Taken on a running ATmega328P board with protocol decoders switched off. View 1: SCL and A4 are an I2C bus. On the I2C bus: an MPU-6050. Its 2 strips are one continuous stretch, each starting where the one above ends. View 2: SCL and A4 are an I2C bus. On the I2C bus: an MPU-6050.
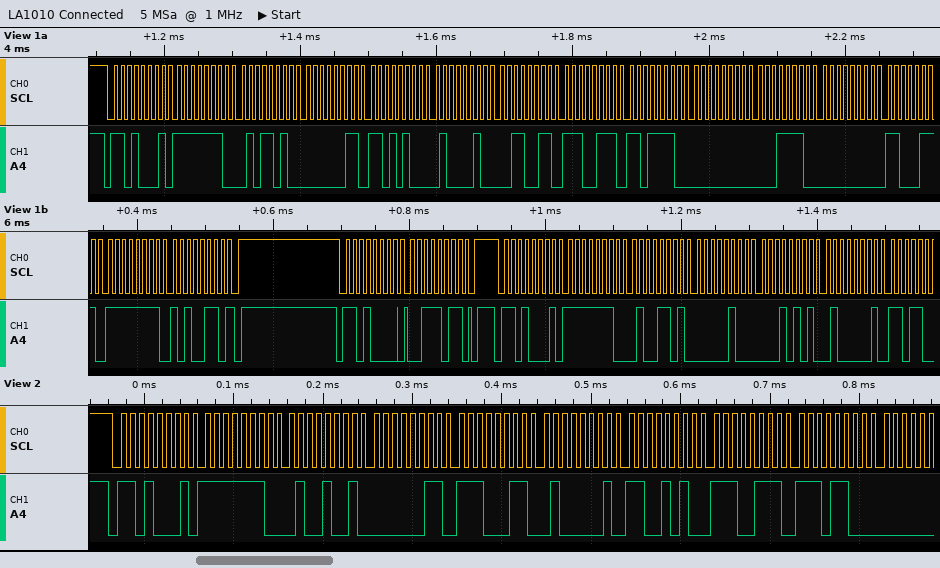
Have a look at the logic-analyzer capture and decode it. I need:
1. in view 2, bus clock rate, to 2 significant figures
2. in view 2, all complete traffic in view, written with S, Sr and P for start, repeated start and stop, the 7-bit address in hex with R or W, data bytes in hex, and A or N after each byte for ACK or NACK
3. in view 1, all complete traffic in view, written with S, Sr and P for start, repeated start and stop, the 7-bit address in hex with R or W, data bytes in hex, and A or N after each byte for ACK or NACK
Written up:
100 kHz
S 68R A FE A 49 A 03 A E3 A 41 A CA A E7 A EC A
S 68R A FE A 5A A 03 A D4 A 42 A 33 A E7 A DE A 00 A 1E A 00 A C7 A FF A A6 N P S 68W A 3B A P S 68R A FE A 4D A 04 A 15 A 41 A
